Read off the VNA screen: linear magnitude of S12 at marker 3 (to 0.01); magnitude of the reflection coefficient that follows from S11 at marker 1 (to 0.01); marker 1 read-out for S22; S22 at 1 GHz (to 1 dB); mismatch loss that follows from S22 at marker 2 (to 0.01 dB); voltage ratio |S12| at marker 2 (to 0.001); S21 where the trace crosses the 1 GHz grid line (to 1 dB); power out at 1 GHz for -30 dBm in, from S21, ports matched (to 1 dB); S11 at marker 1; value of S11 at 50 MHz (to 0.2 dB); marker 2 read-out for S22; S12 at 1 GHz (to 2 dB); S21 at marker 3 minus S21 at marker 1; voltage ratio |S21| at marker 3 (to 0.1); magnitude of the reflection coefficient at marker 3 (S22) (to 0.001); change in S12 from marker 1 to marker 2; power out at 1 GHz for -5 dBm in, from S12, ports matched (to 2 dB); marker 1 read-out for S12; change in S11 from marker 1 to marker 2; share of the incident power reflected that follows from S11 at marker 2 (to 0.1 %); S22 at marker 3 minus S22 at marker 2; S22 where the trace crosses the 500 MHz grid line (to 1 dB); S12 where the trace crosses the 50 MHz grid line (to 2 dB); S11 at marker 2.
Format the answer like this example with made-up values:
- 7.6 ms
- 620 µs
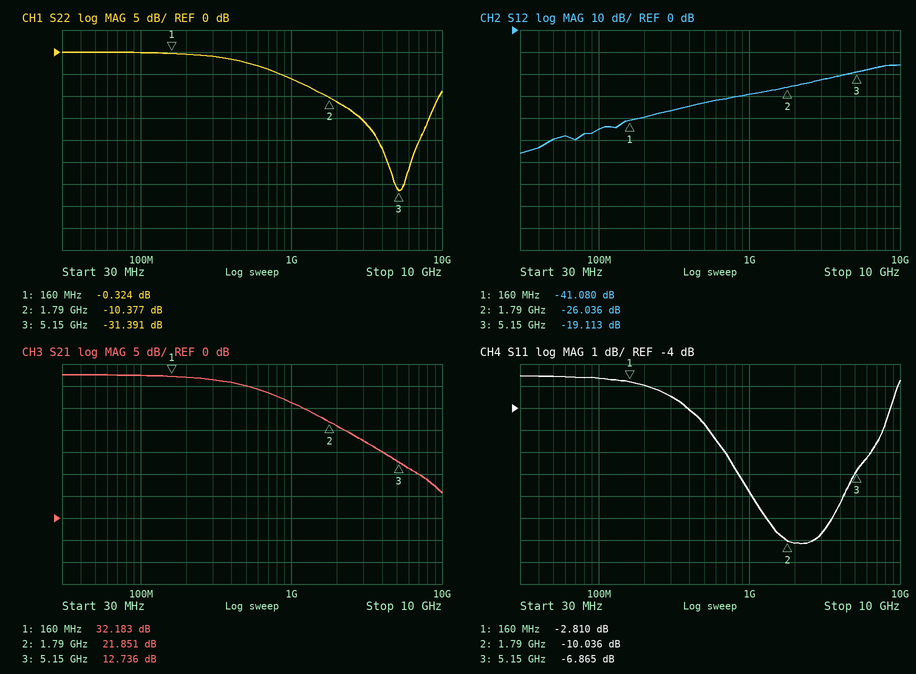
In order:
- 0.11
- 0.72
- -0.324 dB
- -6 dB
- 0.42 dB
- 0.050
- 26 dB
- -4 dBm
- -2.810 dB
- -2.6 dB
- -10.377 dB
- -30 dB
- -19.447 dB
- 4.3
- 0.027
- 15.044 dB
- -34 dBm
- -41.080 dB
- -7.226 dB
- 9.9 %
- -21.014 dB
- -2 dB
- -50 dB
- -10.036 dB
